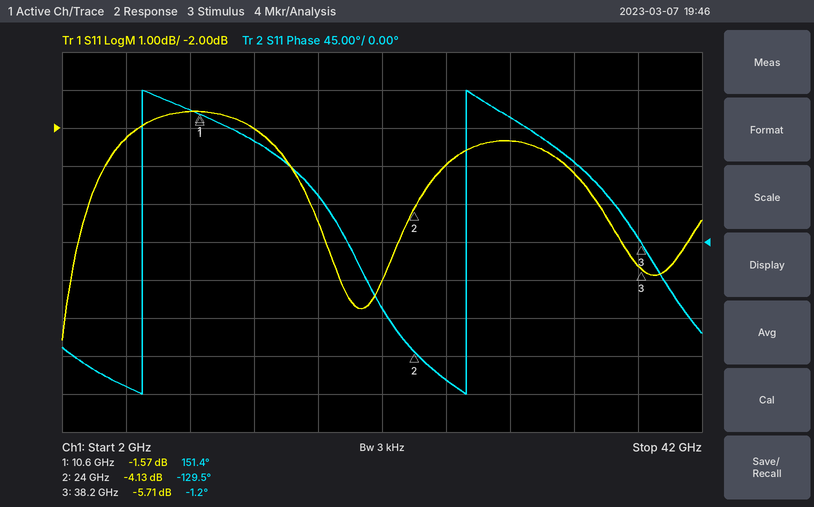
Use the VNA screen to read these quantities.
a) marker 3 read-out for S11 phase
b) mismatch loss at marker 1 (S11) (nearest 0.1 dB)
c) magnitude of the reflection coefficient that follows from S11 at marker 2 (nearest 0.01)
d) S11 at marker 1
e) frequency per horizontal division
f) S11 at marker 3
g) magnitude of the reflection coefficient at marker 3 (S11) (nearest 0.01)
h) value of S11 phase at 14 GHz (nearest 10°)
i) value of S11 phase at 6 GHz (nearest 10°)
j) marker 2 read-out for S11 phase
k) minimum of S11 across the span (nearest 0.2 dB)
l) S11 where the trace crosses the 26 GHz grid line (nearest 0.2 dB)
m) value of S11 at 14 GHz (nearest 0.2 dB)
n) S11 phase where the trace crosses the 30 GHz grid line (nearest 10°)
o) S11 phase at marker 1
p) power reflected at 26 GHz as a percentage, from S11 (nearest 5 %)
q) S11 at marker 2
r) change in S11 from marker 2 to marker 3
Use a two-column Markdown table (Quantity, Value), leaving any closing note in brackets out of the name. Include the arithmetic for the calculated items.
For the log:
| Quantity | Value |
|---|---|
| marker 3 read-out for S11 phase | -1.2° |
| mismatch loss at marker 1 (S11) | −10 log10(1 − 10^(-1.57/10)) ≈ 5.2 dB |
| magnitude of the reflection coefficient that follows from S11 at marker 2 | 10^(-4.13/20) ≈ 0.62 |
| S11 at marker 1 | -1.57 dB |
| frequency per horizontal division | 4 GHz |
| S11 at marker 3 | -5.71 dB |
| magnitude of the reflection coefficient at marker 3 (S11) | 10^(-5.71/20) ≈ 0.52 |
| value of S11 phase at 14 GHz | 120° |
| value of S11 phase at 6 GHz | -170° |
| marker 2 read-out for S11 phase | -129.5° |
| minimum of S11 across the span | -7.6 dB |
| S11 where the trace crosses the 26 GHz grid line | -3.0 dB |
| value of S11 at 14 GHz | -2.0 dB |
| S11 phase where the trace crosses the 30 GHz grid line | 150° |
| S11 phase at marker 1 | 151.4° |
| power reflected at 26 GHz as a percentage, from S11 | 10^(-3/10) ≈ 50 % |
| S11 at marker 2 | -4.13 dB |
| change in S11 from marker 2 to marker 3 | -5.71 − (-4.13) = -1.58 dB |
